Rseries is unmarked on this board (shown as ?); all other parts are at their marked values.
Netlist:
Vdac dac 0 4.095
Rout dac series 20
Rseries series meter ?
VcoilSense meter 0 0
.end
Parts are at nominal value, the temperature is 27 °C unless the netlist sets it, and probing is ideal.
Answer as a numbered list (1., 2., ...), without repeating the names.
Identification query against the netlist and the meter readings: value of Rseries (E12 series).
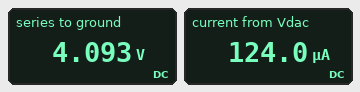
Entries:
1. 33 kΩ
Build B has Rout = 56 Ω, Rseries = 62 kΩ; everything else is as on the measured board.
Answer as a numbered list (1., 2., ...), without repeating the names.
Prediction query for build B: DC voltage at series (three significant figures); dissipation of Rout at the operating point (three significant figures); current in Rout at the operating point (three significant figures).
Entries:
1. 4.09 V
2. 244 nW
3. 66.0 µA
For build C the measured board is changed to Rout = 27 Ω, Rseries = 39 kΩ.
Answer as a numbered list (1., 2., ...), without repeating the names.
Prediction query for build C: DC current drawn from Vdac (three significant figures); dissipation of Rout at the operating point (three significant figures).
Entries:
1. 105 µA
2. 297 nW
